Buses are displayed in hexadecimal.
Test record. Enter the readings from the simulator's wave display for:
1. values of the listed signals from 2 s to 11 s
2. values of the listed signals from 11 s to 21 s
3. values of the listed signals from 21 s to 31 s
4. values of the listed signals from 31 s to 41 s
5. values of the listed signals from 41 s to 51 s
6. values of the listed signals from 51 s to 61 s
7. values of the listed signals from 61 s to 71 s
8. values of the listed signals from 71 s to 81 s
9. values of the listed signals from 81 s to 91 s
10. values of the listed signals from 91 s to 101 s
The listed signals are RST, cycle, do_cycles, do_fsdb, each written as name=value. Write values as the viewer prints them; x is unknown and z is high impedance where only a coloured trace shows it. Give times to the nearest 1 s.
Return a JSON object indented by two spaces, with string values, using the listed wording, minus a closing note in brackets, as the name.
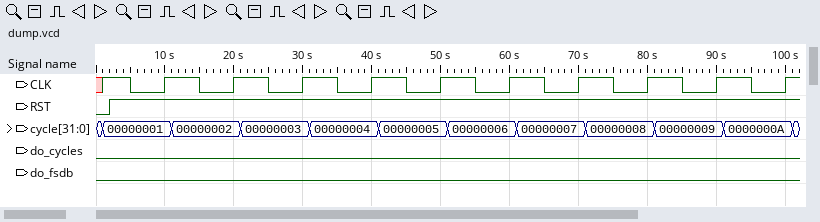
{
  "values of the listed signals from 2 s to 11 s": "RST=1, cycle=00000001, do_cycles=0, do_fsdb=0",
  "values of the listed signals from 11 s to 21 s": "RST=1, cycle=00000002, do_cycles=0, do_fsdb=0",
  "values of the listed signals from 21 s to 31 s": "RST=1, cycle=00000003, do_cycles=0, do_fsdb=0",
  "values of the listed signals from 31 s to 41 s": "RST=1, cycle=00000004, do_cycles=0, do_fsdb=0",
  "values of the listed signals from 41 s to 51 s": "RST=1, cycle=00000005, do_cycles=0, do_fsdb=0",
  "values of the listed signals from 51 s to 61 s": "RST=1, cycle=00000006, do_cycles=0, do_fsdb=0",
  "values of the listed signals from 61 s to 71 s": "RST=1, cycle=00000007, do_cycles=0, do_fsdb=0",
  "values of the listed signals from 71 s to 81 s": "RST=1, cycle=00000008, do_cycles=0, do_fsdb=0",
  "values of the listed signals from 81 s to 91 s": "RST=1, cycle=00000009, do_cycles=0, do_fsdb=0",
  "values of the listed signals from 91 s to 101 s": "RST=1, cycle=0000000A, do_cycles=0, do_fsdb=0"
}
